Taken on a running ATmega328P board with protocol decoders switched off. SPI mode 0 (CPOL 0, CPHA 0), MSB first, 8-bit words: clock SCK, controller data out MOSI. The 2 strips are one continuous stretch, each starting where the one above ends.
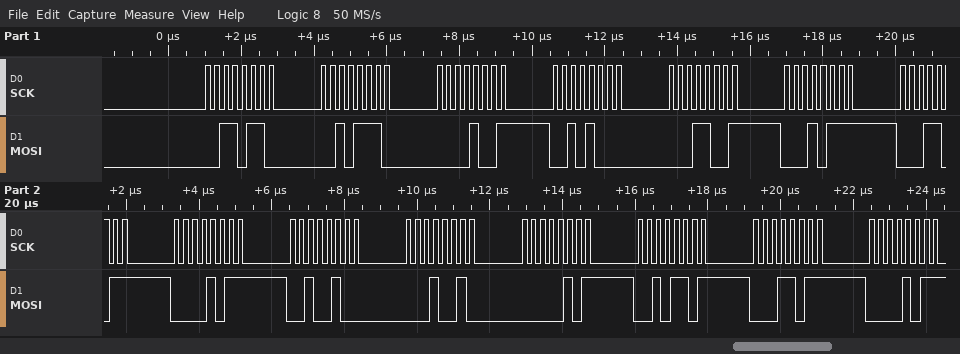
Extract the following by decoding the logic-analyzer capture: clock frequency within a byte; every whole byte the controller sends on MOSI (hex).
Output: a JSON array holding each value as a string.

["4 MHz", "36 2E 09 28 19 17 1B 0B 24 12 05 2D 1B 0B"]
